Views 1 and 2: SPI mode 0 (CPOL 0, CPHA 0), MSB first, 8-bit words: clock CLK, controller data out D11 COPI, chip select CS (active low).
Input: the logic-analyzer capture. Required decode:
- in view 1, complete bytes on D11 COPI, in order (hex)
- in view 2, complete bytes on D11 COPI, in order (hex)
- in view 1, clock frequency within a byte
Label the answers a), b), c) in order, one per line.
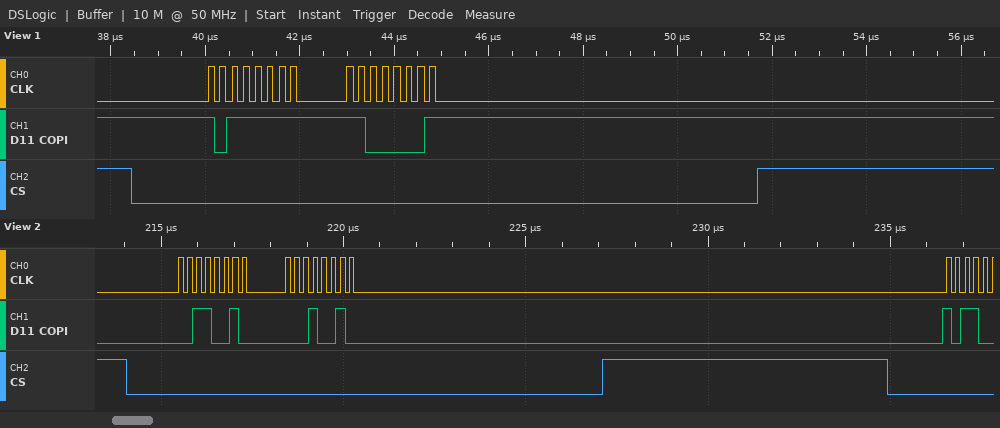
a) BF C1
b) 32 12
c) 4 MHz
